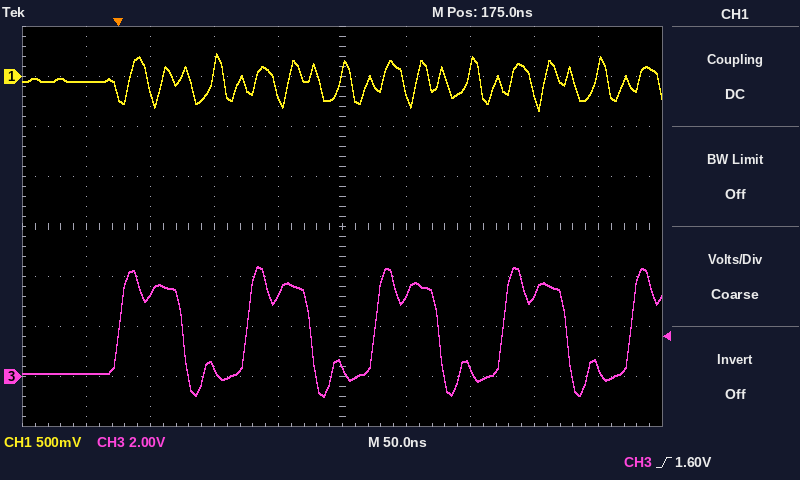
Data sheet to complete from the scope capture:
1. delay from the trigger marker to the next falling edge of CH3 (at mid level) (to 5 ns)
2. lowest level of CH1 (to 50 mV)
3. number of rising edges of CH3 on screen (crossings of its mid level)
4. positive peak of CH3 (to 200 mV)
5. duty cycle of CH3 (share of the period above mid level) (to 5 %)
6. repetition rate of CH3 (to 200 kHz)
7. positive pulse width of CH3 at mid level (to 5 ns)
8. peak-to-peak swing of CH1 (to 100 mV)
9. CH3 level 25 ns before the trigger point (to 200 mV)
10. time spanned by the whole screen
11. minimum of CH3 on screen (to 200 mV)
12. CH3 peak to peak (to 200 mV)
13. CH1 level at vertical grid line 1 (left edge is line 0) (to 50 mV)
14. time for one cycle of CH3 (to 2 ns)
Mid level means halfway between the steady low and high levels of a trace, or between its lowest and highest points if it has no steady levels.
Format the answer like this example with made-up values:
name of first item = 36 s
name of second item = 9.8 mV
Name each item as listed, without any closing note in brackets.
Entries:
delay from the trigger marker to the next falling edge of CH3 (at mid level) = 50 ns
lowest level of CH1 = -350 mV
number of rising edges of CH3 on screen = 5
positive peak of CH3 = 4.4 V
duty cycle of CH3 (share of the period above mid level) = 50 %
repetition rate of CH3 = 10.0 MHz
positive pulse width of CH3 at mid level = 50 ns
peak-to-peak swing of CH1 = 600 mV
CH3 level 25 ns before the trigger point = 200 mV
time spanned by the whole screen = 500 ns
minimum of CH3 on screen = -800 mV
CH3 peak to peak = 5.2 V
CH1 level at vertical grid line 1 (left edge is line 0) = -50 mV
time for one cycle of CH3 = 100 ns
